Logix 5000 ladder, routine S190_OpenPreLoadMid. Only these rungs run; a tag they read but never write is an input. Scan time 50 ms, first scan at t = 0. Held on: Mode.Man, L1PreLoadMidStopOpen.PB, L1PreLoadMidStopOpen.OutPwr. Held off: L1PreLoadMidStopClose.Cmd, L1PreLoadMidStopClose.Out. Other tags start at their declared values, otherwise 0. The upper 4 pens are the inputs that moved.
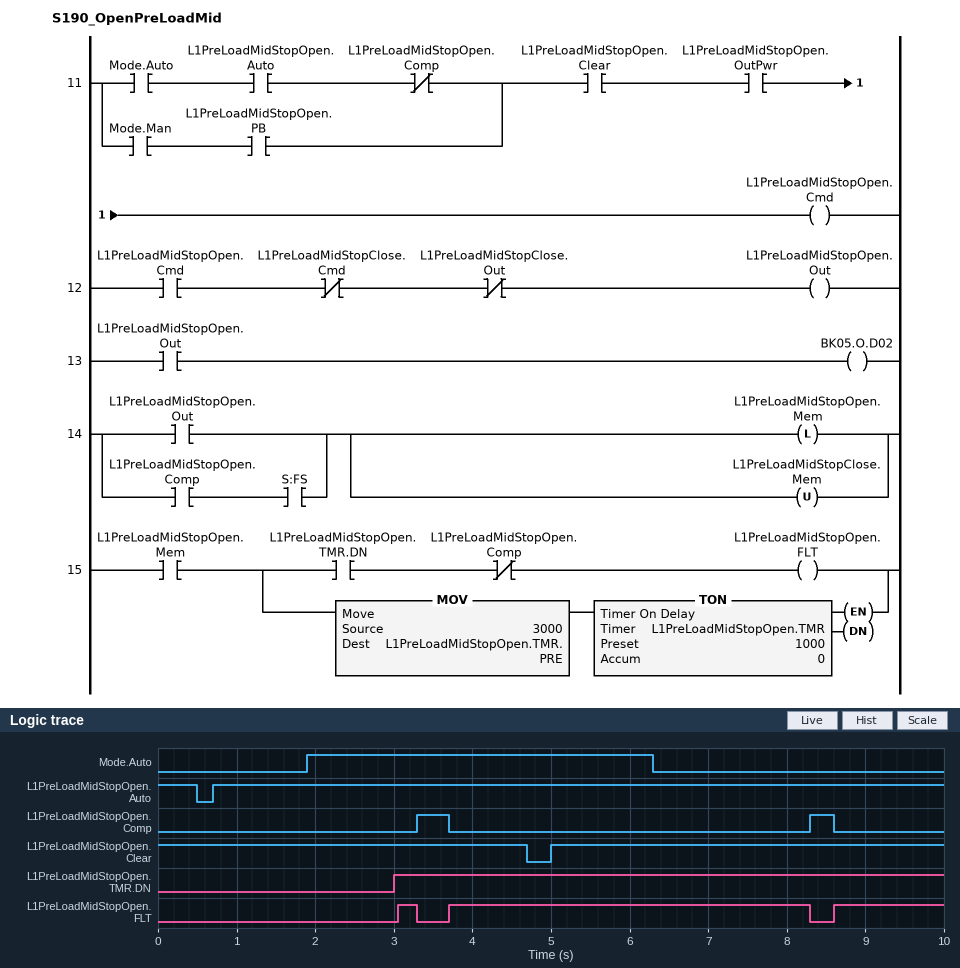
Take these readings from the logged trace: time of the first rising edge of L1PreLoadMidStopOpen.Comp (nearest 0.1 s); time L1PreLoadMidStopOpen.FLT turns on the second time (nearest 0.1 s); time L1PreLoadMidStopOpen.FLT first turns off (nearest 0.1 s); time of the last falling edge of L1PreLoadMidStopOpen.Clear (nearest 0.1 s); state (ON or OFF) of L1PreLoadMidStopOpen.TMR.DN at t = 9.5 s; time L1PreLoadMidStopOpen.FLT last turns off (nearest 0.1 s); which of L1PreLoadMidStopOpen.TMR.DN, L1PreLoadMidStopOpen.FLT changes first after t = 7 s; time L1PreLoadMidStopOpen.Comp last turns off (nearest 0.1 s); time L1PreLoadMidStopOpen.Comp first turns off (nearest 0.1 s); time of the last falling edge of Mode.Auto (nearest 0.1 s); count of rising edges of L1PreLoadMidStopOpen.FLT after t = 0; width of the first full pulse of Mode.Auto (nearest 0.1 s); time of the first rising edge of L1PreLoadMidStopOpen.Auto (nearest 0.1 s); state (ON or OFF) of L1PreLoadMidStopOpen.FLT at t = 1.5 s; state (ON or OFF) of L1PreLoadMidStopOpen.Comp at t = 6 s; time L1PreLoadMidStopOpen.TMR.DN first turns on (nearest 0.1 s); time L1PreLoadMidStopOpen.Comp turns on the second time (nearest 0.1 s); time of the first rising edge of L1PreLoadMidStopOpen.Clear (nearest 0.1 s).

3.3 s
3.7 s
3.3 s
4.7 s
ON
8.3 s
L1PreLoadMidStopOpen.FLT
8.6 s
3.7 s
6.3 s
3
4.4 s
0.7 s
OFF
OFF
3.0 s
8.3 s
5.0 s
